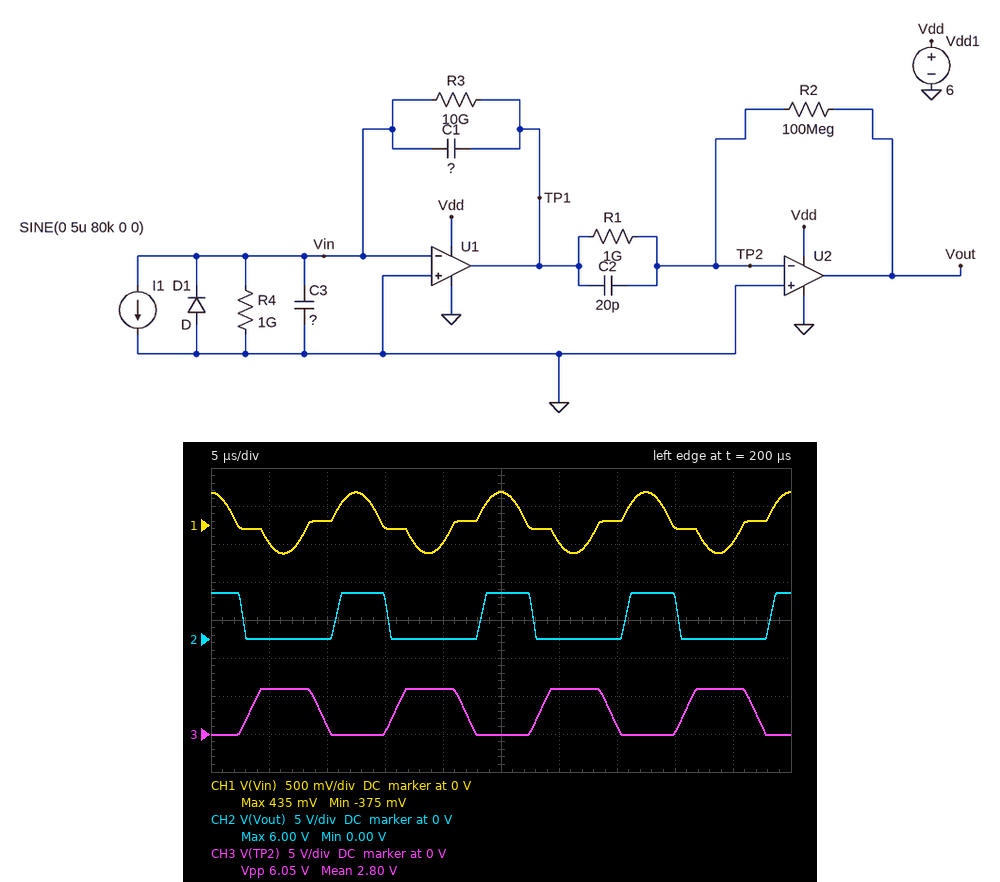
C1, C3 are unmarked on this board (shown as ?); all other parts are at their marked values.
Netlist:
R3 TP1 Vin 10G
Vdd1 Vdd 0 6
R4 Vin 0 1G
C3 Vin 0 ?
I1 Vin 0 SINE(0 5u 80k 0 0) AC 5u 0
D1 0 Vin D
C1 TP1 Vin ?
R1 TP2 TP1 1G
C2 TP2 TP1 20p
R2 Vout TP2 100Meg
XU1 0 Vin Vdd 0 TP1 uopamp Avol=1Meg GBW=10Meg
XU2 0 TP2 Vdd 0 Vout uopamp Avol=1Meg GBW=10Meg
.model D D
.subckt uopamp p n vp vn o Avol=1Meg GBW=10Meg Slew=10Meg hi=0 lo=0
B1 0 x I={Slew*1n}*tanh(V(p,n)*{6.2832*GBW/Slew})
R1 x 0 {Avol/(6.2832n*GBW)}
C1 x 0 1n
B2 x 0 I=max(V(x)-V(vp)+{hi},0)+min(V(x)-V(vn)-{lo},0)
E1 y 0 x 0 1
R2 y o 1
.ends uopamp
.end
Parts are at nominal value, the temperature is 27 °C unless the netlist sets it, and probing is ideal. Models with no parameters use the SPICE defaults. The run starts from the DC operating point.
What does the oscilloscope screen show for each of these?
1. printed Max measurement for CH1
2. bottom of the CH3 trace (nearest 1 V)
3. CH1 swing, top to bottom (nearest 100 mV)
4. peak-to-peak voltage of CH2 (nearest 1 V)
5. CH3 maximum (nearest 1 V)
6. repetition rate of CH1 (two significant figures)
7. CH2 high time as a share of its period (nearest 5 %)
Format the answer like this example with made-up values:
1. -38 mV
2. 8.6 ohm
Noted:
1. 435 mV
2. 0 V
3. 800 mV
4. 6 V
5. 6 V
6. 80 kHz
7. 35 %
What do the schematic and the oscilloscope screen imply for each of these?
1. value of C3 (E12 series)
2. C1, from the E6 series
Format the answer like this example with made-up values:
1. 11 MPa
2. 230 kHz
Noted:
1. 12 pF
2. 1.5 pF
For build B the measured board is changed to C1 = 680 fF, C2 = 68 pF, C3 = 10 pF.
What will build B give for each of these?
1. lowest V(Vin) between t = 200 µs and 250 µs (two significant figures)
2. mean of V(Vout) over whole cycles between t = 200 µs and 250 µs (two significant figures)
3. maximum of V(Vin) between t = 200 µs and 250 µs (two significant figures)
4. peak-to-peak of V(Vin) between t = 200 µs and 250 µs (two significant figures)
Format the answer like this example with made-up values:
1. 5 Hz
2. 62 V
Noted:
1. -380 mV
2. 2.2 V
3. 1.1 V
4. 1.5 V
